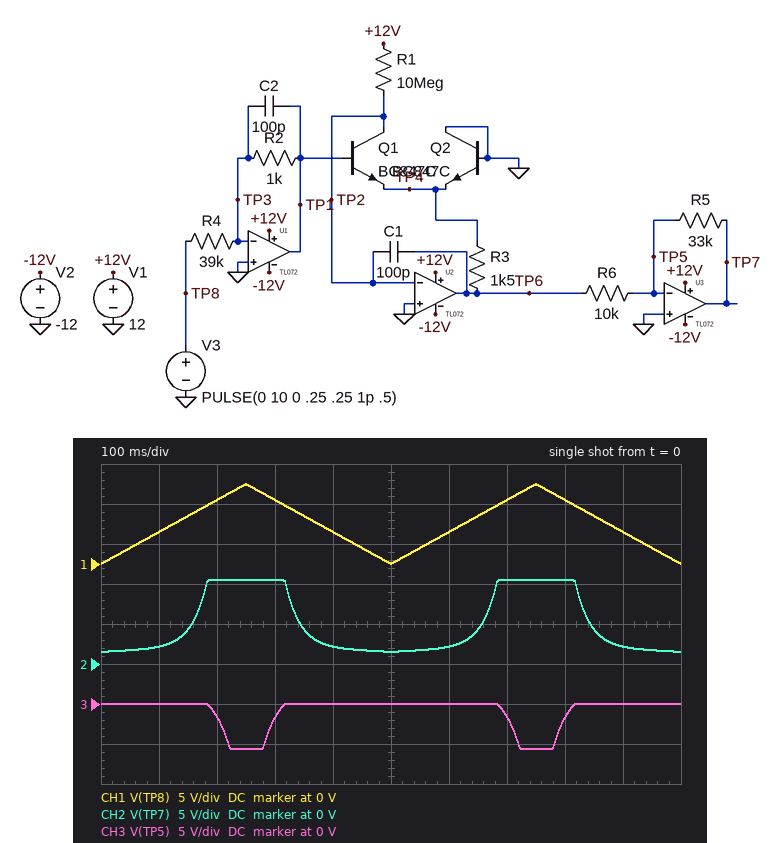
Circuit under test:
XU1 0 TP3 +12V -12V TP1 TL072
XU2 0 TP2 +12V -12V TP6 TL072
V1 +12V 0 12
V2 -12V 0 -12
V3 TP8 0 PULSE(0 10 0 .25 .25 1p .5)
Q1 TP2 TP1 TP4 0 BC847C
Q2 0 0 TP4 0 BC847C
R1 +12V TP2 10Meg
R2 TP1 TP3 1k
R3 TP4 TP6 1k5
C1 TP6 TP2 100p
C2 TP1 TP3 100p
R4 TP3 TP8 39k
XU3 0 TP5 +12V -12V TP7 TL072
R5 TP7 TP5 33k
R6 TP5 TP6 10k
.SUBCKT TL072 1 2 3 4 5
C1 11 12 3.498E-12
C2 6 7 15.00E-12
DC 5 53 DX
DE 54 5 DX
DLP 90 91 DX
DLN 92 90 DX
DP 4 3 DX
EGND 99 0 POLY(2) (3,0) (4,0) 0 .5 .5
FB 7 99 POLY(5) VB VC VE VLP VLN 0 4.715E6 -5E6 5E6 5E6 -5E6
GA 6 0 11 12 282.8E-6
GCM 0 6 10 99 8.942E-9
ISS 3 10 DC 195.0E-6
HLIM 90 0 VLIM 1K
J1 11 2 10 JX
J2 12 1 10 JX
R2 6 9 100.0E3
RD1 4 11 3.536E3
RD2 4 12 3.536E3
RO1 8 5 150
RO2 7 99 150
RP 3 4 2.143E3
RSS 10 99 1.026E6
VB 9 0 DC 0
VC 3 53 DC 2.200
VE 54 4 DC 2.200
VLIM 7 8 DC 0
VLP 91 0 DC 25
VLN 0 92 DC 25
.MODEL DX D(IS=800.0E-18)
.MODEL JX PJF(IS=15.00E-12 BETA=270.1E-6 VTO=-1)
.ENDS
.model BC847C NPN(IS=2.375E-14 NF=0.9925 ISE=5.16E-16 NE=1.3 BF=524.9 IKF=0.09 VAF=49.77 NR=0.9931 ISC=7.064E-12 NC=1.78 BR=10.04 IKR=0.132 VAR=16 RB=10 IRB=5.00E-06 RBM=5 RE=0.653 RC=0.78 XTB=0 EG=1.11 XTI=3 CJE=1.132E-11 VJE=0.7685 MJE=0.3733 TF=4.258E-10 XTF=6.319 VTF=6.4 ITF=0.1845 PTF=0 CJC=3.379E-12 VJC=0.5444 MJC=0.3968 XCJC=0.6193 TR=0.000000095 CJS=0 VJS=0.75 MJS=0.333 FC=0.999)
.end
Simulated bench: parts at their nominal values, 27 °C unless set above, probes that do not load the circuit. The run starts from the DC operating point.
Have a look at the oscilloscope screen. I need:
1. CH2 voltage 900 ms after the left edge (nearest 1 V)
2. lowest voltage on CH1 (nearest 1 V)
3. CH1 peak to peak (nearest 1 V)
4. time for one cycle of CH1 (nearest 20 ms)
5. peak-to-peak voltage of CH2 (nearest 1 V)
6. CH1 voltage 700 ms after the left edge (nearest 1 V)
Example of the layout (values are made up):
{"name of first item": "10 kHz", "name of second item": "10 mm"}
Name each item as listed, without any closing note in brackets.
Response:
{"CH2 voltage 900 ms after the left edge": "2 V", "lowest voltage on CH1": "0 V", "CH1 peak to peak": "10 V", "time for one cycle of CH1": "500 ms", "peak-to-peak voltage of CH2": "9 V", "CH1 voltage 700 ms after the left edge": "8 V"}
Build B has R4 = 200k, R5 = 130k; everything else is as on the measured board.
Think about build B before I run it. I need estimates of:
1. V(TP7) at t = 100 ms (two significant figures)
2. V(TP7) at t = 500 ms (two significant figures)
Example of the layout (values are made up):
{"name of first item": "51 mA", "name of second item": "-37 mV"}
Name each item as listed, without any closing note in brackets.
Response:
{"V(TP7) at t = 100 ms": "6.3 V", "V(TP7) at t = 500 ms": "6.0 V"}
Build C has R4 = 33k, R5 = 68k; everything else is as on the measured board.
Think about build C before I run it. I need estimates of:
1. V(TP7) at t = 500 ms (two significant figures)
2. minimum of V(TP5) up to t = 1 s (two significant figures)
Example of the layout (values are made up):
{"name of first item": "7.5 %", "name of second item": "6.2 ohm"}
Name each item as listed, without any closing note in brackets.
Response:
{"V(TP7) at t = 500 ms": "3.1 V", "minimum of V(TP5) up to t = 1 s": "-7.8 V"}
